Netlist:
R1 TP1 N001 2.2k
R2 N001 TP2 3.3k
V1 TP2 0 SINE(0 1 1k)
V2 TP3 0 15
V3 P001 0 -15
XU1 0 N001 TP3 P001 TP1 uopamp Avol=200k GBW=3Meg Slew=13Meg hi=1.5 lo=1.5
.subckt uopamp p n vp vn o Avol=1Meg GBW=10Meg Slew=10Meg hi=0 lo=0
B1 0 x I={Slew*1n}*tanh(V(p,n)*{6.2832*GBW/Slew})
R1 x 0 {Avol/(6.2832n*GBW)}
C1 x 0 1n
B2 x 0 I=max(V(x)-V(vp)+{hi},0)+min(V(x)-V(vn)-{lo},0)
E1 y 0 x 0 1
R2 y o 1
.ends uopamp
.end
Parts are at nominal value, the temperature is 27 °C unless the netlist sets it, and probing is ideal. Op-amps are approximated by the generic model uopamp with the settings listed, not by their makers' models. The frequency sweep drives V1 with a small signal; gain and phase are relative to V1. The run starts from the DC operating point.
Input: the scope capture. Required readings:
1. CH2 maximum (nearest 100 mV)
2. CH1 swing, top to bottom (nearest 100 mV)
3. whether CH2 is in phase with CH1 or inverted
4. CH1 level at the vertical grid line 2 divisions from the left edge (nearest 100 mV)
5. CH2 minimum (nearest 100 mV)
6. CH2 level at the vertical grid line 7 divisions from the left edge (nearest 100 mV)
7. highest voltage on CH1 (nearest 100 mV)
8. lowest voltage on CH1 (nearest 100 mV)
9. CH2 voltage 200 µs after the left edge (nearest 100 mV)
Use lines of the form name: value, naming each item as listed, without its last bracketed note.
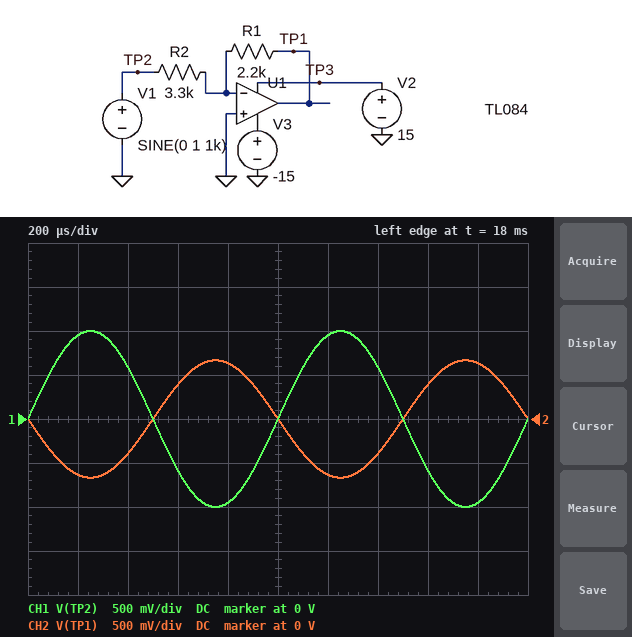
CH2 maximum: 700 mV
CH1 swing, top to bottom: 2.0 V
whether CH2 is in phase with CH1 or inverted: inverted
CH1 level at the vertical grid line 2 divisions from the left edge: 600 mV
CH2 minimum: -700 mV
CH2 level at the vertical grid line 7 divisions from the left edge: -400 mV
highest voltage on CH1: 1.0 V
lowest voltage on CH1: -1.0 V
CH2 voltage 200 µs after the left edge: -600 mV
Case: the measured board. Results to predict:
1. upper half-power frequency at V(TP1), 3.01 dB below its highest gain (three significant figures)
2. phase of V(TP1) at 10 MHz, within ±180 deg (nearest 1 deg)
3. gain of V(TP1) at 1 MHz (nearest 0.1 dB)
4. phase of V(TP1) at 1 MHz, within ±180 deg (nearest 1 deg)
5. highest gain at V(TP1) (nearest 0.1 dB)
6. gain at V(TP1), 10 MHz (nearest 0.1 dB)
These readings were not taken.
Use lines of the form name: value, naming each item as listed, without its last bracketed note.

upper half-power frequency at V(TP1), 3.01 dB below its highest gain: 1.80 MHz
phase of V(TP1) at 10 MHz, within ±180 deg: 100 deg
gain of V(TP1) at 1 MHz: -4.7 dB
phase of V(TP1) at 1 MHz, within ±180 deg: 151 deg
highest gain at V(TP1): -3.5 dB
gain at V(TP1), 10 MHz: -18.6 dB
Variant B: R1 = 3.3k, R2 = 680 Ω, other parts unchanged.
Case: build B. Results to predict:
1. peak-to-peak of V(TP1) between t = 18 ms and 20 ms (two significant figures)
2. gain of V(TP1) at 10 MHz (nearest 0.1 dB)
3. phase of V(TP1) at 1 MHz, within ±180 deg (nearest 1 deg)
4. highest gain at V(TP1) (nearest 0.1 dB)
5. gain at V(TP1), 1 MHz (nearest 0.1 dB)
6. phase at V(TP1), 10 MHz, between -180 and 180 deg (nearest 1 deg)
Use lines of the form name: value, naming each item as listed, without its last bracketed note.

peak-to-peak of V(TP1) between t = 18 ms and 20 ms: 9.7 V
gain of V(TP1) at 10 MHz: -12.1 dB
phase of V(TP1) at 1 MHz, within ±180 deg: 117 deg
highest gain at V(TP1): 13.7 dB
gain at V(TP1), 1 MHz: 6.9 dB
phase at V(TP1), 10 MHz, between -180 and 180 deg: 93 deg
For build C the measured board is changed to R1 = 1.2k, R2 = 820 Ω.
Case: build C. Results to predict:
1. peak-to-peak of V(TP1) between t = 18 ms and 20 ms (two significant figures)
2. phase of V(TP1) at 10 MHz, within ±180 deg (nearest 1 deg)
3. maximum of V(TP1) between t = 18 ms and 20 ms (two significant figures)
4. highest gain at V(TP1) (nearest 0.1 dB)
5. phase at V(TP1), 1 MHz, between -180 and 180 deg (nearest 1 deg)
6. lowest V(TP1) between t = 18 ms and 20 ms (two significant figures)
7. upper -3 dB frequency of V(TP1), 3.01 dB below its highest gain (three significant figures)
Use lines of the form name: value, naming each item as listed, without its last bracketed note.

peak-to-peak of V(TP1) between t = 18 ms and 20 ms: 2.9 V
phase of V(TP1) at 10 MHz, within ±180 deg: 97 deg
maximum of V(TP1) between t = 18 ms and 20 ms: 1.5 V
highest gain at V(TP1): 3.3 dB
phase at V(TP1), 1 MHz, between -180 and 180 deg: 141 deg
lowest V(TP1) between t = 18 ms and 20 ms: -1.5 V
upper -3 dB frequency of V(TP1), 3.01 dB below its highest gain: 1.22 MHz
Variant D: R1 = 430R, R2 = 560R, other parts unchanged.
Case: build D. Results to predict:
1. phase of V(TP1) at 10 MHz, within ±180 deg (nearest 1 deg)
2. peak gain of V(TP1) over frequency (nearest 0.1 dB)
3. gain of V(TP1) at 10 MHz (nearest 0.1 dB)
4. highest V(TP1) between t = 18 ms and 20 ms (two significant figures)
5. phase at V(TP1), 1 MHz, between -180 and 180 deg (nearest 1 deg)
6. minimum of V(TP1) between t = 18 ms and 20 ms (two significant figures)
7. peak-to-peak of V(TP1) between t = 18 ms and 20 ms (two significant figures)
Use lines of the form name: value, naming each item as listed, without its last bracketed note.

phase of V(TP1) at 10 MHz, within ±180 deg: 99 deg
peak gain of V(TP1) over frequency: -2.3 dB
gain of V(TP1) at 10 MHz: -17.8 dB
highest V(TP1) between t = 18 ms and 20 ms: 770 mV
phase at V(TP1), 1 MHz, between -180 and 180 deg: 149 deg
minimum of V(TP1) between t = 18 ms and 20 ms: -770 mV
peak-to-peak of V(TP1) between t = 18 ms and 20 ms: 1.5 V
